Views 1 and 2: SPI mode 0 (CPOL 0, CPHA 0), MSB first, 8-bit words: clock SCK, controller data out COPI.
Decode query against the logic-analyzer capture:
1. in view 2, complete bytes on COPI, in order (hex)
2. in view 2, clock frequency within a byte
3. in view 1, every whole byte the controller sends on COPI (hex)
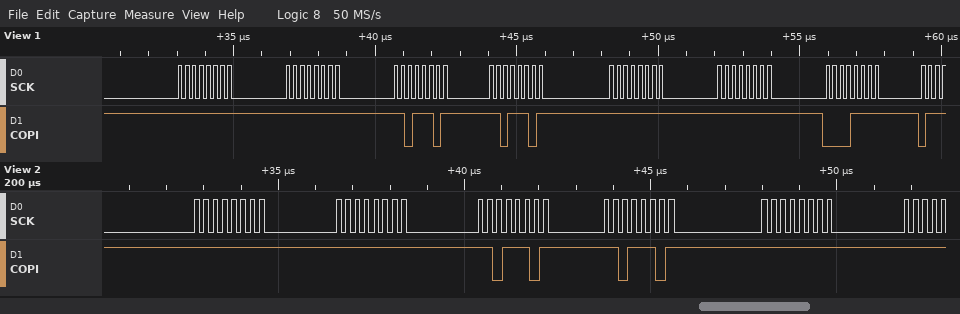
FF FF DD DD FF
4 MHz
FF FF DD DD FF FF 0F
